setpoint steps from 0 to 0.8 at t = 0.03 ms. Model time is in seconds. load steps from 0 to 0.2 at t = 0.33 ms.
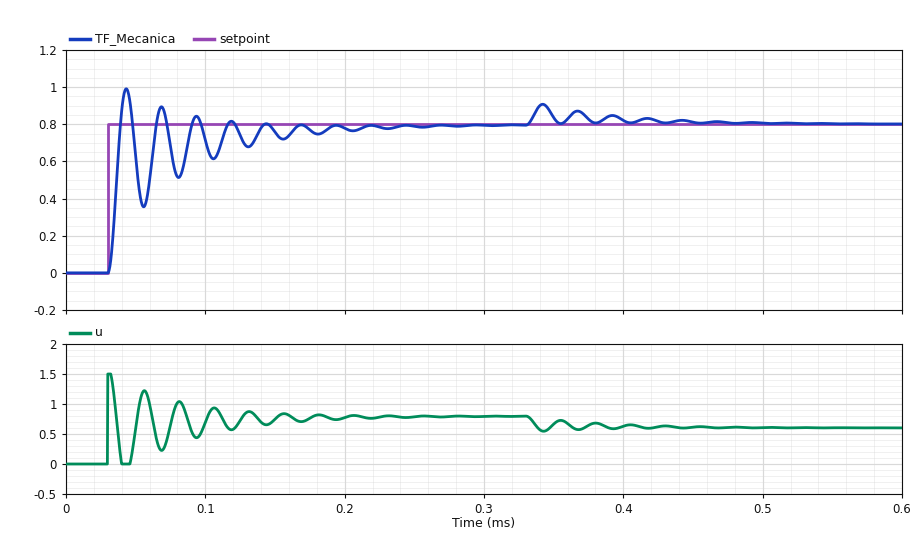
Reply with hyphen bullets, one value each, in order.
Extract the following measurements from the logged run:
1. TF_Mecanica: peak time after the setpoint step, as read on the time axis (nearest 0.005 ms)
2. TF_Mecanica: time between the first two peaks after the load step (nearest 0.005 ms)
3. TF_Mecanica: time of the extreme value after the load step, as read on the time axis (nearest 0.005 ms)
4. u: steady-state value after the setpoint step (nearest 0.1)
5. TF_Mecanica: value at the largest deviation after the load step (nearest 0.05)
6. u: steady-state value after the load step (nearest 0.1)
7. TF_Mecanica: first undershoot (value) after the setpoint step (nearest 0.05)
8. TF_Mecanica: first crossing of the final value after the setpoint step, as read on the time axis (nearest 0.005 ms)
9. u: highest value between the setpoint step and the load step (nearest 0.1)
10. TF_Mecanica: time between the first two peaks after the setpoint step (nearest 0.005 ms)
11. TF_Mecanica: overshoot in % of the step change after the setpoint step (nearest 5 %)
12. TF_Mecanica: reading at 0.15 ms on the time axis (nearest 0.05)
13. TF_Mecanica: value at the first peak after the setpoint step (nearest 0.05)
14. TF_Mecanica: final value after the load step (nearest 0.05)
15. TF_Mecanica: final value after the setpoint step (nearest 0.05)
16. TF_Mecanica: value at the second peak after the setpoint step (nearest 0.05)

- 0.045 ms
- 0.025 ms
- 0.340 ms
- 0.8
- 0.90
- 0.6
- 0.35
- 0.040 ms
- 1.5
- 0.025 ms
- 25 %
- 0.75
- 1.00
- 0.80
- 0.80
- 0.90
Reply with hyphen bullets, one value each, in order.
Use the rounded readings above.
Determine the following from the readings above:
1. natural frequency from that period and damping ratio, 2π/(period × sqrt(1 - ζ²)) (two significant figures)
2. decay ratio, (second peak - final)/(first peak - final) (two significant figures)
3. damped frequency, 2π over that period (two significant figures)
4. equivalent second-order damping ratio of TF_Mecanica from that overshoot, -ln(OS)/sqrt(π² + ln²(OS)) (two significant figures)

- 270 rad/ms
- 0.50
- 250 rad/ms
- 0.40
